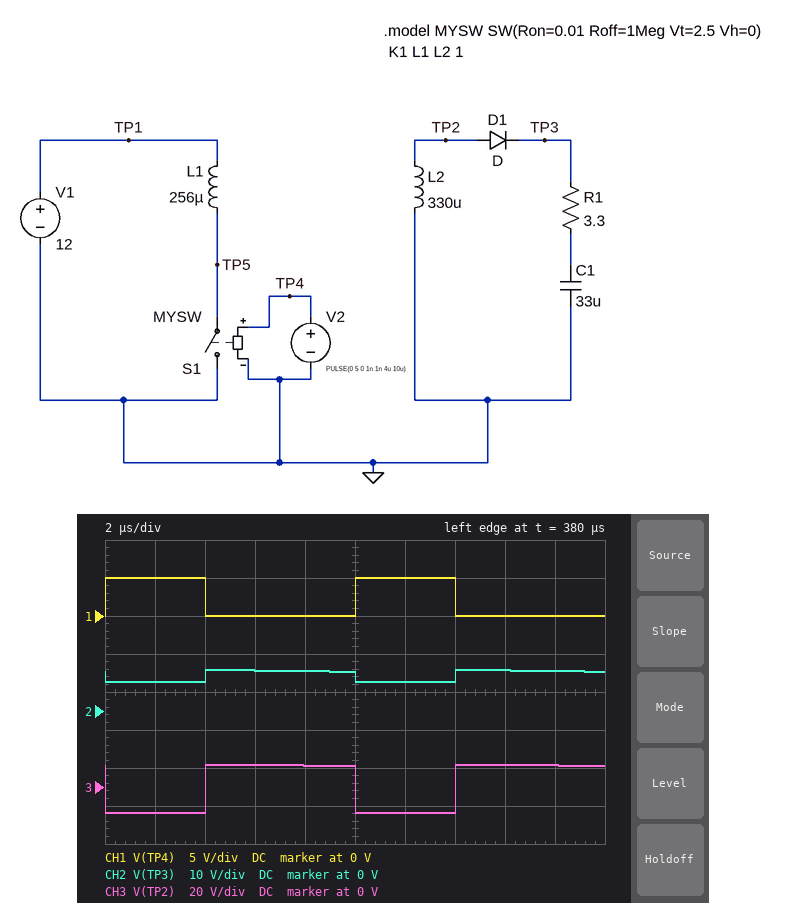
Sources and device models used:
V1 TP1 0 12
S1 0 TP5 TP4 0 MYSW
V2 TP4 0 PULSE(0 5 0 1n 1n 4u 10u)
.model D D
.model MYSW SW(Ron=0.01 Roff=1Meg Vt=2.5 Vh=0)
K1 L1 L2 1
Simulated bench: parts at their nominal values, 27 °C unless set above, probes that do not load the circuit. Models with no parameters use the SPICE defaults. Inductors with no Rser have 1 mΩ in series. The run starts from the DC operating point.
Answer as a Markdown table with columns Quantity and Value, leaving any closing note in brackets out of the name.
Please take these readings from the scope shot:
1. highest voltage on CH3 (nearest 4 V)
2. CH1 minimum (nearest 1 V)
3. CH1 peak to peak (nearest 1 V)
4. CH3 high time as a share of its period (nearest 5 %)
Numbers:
| Quantity | Value |
|---|---|
| highest voltage on CH3 | 12 V |
| CH1 minimum | 0 V |
| CH1 peak to peak | 5 V |
| CH3 high time as a share of its period | 60 % |
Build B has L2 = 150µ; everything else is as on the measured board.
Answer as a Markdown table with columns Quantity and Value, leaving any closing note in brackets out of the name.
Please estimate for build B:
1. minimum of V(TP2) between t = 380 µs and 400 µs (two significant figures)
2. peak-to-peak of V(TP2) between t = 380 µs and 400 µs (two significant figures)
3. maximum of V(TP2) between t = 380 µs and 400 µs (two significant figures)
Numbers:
| Quantity | Value |
|---|---|
| minimum of V(TP2) between t = 380 µs and 400 µs | -9.2 V |
| peak-to-peak of V(TP2) between t = 380 µs and 400 µs | 16 V |
| maximum of V(TP2) between t = 380 µs and 400 µs | 7.2 V |
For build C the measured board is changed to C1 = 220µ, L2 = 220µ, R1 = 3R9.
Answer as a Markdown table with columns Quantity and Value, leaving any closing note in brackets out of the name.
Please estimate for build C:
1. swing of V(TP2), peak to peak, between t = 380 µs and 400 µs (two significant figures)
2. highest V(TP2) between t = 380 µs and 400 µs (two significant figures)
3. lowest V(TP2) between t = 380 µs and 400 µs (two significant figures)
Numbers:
| Quantity | Value |
|---|---|
| swing of V(TP2), peak to peak, between t = 380 µs and 400 µs | 19 V |
| highest V(TP2) between t = 380 µs and 400 µs | 8.1 V |
| lowest V(TP2) between t = 380 µs and 400 µs | -11 V |
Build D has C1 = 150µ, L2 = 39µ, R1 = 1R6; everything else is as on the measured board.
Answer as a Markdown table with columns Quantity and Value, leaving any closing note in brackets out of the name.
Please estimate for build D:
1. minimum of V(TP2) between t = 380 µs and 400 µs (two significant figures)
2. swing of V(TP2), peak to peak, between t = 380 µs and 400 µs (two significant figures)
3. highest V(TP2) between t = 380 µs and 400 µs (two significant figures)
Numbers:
| Quantity | Value |
|---|---|
| minimum of V(TP2) between t = 380 µs and 400 µs | -4.7 V |
| swing of V(TP2), peak to peak, between t = 380 µs and 400 µs | 8.3 V |
| highest V(TP2) between t = 380 µs and 400 µs | 3.6 V |
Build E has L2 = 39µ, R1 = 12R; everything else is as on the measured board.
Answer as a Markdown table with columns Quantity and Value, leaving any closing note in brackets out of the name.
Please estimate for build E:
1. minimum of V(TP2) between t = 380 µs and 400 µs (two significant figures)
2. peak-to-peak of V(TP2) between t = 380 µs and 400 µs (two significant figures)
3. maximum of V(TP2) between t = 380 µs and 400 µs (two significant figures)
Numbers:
| Quantity | Value |
|---|---|
| minimum of V(TP2) between t = 380 µs and 400 µs | -4.7 V |
| peak-to-peak of V(TP2) between t = 380 µs and 400 µs | 12 V |
| maximum of V(TP2) between t = 380 µs and 400 µs | 7.7 V |
